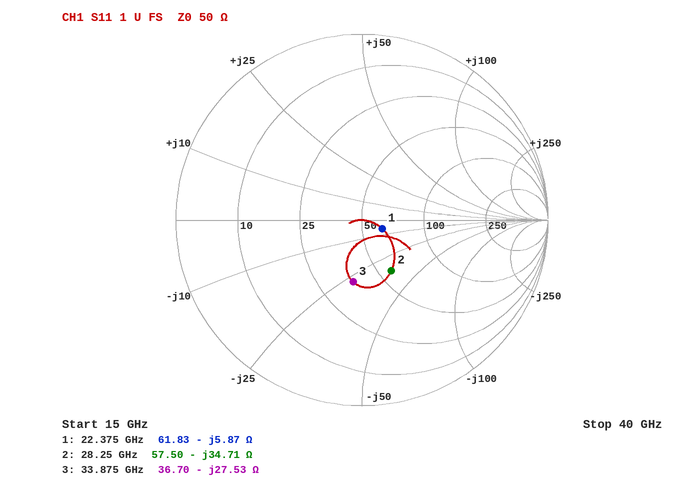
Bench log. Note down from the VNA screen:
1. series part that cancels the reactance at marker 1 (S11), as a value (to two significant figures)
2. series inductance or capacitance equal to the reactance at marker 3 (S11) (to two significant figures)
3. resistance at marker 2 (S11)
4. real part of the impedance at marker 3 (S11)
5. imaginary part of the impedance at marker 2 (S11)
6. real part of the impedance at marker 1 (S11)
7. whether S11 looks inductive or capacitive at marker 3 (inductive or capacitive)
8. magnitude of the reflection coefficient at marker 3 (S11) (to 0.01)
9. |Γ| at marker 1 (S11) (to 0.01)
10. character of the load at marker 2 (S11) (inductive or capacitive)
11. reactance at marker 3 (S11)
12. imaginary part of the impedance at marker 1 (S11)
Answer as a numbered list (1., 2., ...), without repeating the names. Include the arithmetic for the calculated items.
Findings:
1. L = 5.87 Ω/(2π × 22.375 GHz) ≈ 42 pH
2. C = 1/(2π × 33.875 GHz × 27.53 Ω) ≈ 171 fF, so 170 fF to two significant figures
3. 57.50 Ω
4. 36.70 Ω
5. -34.71 Ω
6. 61.83 Ω
7. capacitive
8. 0.34
9. 0.12
10. capacitive
11. -27.53 Ω
12. -5.87 Ω
